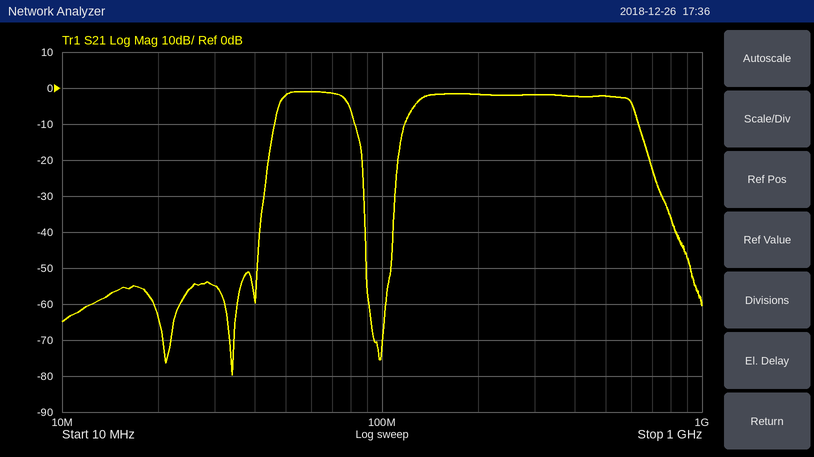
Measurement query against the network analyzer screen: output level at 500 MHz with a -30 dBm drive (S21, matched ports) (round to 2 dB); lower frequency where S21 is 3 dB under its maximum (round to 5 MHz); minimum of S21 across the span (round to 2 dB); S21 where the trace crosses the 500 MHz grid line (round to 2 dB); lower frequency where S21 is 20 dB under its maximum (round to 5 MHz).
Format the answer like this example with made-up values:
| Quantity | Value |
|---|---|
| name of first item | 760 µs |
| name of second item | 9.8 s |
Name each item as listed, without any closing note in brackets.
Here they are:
| Quantity | Value |
|---|---|
| output level at 500 MHz with a -30 dBm drive (S21, matched ports) | -32 dBm |
| lower frequency where S21 is 3 dB under its maximum | 50 MHz |
| minimum of S21 across the span | -80 dB |
| S21 where the trace crosses the 500 MHz grid line | -2 dB |
| lower frequency where S21 is 20 dB under its maximum | 45 MHz |
